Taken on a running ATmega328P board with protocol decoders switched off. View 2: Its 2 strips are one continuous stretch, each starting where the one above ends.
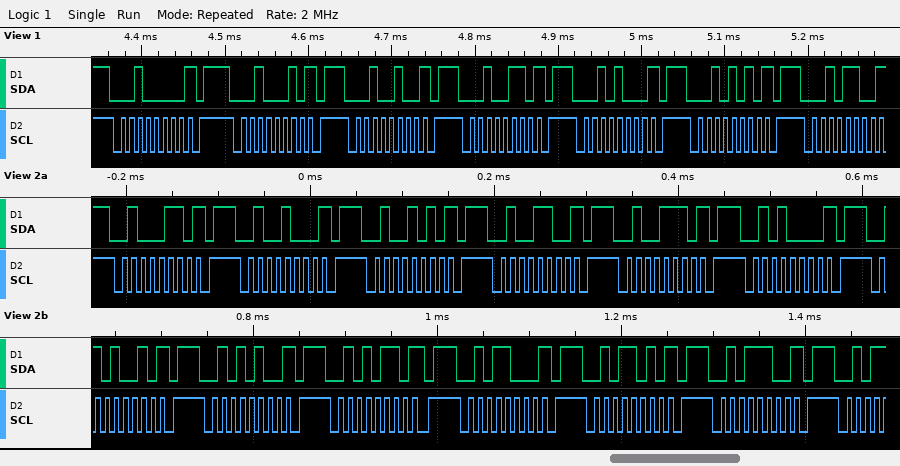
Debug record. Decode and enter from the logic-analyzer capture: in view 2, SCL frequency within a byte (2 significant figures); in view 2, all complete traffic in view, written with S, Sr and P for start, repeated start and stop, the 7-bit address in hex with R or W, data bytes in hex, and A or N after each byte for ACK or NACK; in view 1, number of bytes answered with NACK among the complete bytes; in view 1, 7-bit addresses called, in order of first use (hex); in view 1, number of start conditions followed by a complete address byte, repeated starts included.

100 kHz
S 23W N P S 24W N P S 25W N P S 26W N P S 27W N P S 28W N P S 29W N P S 2AW N P S 2BW N P S 2CW N P S 2DW N P S 2EW N P
7
0x10 0x11 0x12 0x13 0x14 0x15 0x16
7
